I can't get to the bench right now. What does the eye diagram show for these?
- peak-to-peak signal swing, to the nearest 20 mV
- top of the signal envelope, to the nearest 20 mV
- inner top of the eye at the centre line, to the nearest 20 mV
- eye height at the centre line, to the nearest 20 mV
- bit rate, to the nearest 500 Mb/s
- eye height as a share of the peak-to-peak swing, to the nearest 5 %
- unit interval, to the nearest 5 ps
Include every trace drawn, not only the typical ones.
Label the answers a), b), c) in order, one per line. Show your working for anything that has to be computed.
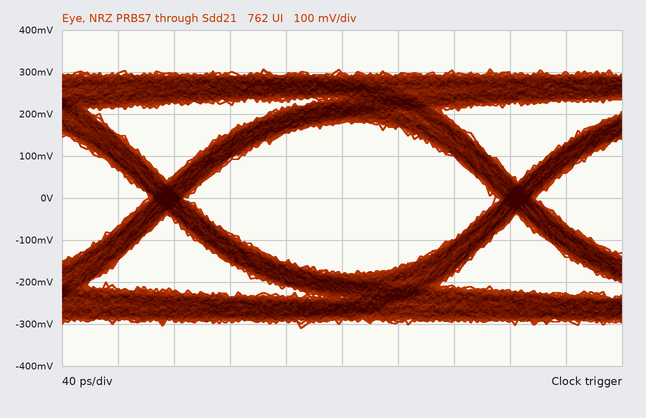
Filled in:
a) 620 mV
b) 300 mV
c) 180 mV
d) 360 mV
e) 4.0 Gb/s
f) 360 mV / 620 mV ≈ 58.1 %, so 60 % to the nearest 5 %
g) 250 ps
